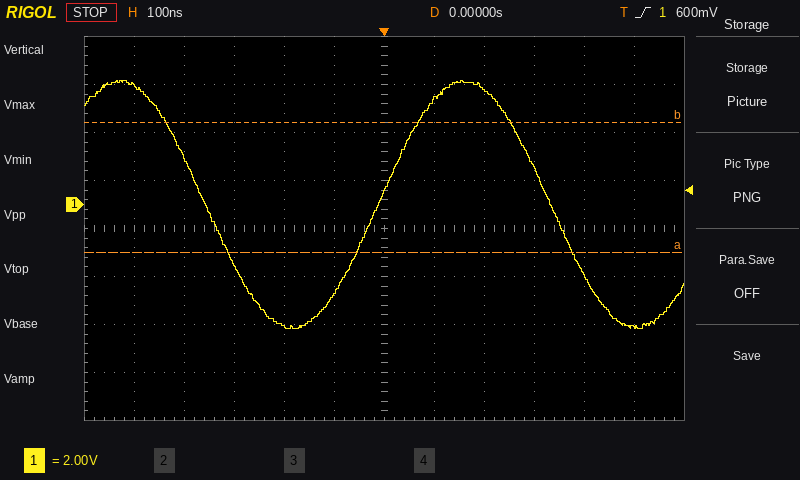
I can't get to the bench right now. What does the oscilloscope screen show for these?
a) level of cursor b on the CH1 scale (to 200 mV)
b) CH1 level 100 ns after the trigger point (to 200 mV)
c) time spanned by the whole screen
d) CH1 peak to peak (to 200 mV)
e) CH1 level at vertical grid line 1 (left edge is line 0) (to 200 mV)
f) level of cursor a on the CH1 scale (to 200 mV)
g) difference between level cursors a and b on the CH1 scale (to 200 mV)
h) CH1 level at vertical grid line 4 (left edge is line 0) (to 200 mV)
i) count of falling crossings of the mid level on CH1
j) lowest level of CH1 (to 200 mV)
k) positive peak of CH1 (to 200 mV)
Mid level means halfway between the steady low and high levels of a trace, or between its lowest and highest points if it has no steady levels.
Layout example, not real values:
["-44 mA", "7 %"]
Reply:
["3.4 V", "4.4 V", "1.2 µs", "10.4 V", "5.0 V", "-2.0 V", "5.4 V", "-5.0 V", "2", "-5.2 V", "5.2 V"]
